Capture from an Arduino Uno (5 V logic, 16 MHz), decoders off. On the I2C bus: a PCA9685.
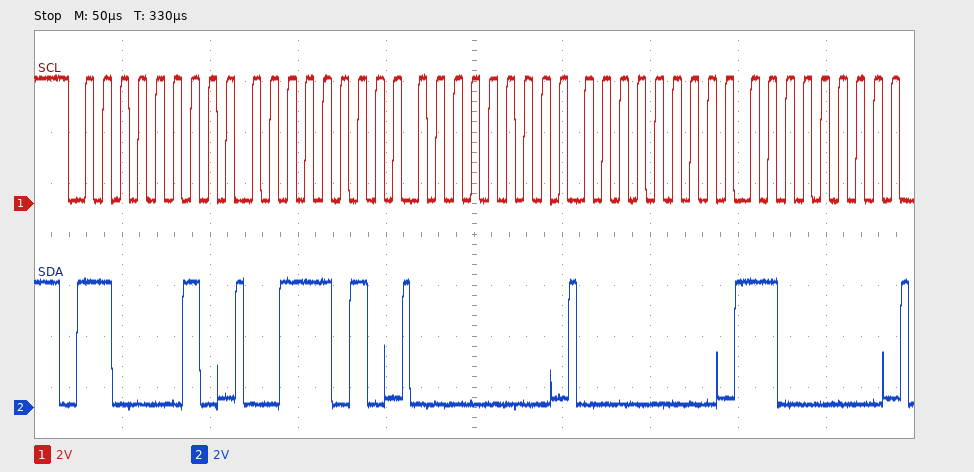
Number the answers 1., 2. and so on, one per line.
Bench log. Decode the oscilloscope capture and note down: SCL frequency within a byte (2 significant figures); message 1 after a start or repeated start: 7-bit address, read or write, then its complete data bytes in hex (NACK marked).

1. 100 kHz
2. 0x61 write: 3A 00 00 C0
